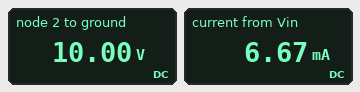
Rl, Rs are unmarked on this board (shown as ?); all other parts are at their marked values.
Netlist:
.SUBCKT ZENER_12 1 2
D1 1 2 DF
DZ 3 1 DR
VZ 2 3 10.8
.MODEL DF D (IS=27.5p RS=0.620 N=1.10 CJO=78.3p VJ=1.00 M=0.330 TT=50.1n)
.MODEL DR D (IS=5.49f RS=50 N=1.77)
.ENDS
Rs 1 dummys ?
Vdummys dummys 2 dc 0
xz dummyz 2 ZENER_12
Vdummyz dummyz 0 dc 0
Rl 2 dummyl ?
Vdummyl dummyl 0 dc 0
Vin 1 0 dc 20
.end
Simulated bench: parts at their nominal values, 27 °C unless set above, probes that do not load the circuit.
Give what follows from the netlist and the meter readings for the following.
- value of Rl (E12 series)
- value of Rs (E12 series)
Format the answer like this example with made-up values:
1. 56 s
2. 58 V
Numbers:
1. 1.5 kΩ
2. 1.5 kΩ
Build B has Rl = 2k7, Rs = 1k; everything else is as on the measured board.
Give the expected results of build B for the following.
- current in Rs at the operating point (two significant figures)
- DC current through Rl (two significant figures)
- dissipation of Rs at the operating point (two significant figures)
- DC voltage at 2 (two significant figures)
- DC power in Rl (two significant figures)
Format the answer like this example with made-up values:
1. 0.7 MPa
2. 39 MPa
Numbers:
1. 7.8 mA
2. 4.5 mA
3. 61 mW
4. 12 V
5. 55 mW
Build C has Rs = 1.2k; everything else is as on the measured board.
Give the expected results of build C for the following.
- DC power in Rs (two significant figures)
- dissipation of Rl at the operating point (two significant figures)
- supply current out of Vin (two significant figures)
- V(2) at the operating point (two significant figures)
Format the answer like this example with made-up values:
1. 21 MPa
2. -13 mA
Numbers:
1. 66 mW
2. 82 mW
3. 7.4 mA
4. 11 V
